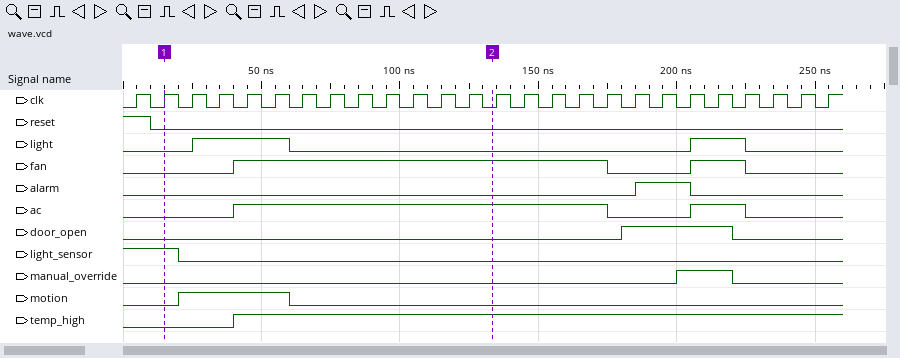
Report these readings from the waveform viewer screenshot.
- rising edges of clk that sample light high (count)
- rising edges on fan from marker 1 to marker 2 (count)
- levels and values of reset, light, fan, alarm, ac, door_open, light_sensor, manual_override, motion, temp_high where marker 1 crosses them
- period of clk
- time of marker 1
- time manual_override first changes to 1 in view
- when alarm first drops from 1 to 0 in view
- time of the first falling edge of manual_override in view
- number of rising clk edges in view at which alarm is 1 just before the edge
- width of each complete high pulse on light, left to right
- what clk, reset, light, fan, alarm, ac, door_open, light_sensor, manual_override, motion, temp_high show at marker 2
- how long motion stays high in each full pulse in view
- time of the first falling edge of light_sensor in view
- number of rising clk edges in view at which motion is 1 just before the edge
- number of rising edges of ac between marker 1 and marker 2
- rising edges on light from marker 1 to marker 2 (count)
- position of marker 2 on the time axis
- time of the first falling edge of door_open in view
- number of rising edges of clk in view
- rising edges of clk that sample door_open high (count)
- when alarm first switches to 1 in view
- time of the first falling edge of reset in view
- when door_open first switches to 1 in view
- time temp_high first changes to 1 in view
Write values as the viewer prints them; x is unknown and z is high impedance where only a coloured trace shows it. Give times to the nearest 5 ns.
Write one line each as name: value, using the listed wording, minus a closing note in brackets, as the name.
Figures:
rising edges of clk that sample light high: 5
rising edges on fan from marker 1 to marker 2: 1
levels and values of reset, light, fan, alarm, ac, door_open, light_sensor, manual_override, motion, temp_high where marker 1 crosses them: reset=0, light=0, fan=0, alarm=0, ac=0, door_open=0, light_sensor=1, manual_override=0, motion=0, temp_high=0
period of clk: 10 ns
time of marker 1: 15 ns
time manual_override first changes to 1 in view: 200 ns
when alarm first drops from 1 to 0 in view: 205 ns
time of the first falling edge of manual_override in view: 220 ns
number of rising clk edges in view at which alarm is 1 just before the edge: 2
width of each complete high pulse on light, left to right: 35 ns, 20 ns
what clk, reset, light, fan, alarm, ac, door_open, light_sensor, manual_override, motion, temp_high show at marker 2: clk=0, reset=0, light=0, fan=1, alarm=0, ac=1, door_open=0, light_sensor=0, manual_override=0, motion=0, temp_high=1
how long motion stays high in each full pulse in view: 40 ns
time of the first falling edge of light_sensor in view: 20 ns
number of rising clk edges in view at which motion is 1 just before the edge: 4
number of rising edges of ac between marker 1 and marker 2: 1
rising edges on light from marker 1 to marker 2: 1
position of marker 2 on the time axis: 135 ns
time of the first falling edge of door_open in view: 220 ns
number of rising edges of clk in view: 26
rising edges of clk that sample door_open high: 4
when alarm first switches to 1 in view: 185 ns
time of the first falling edge of reset in view: 10 ns
when door_open first switches to 1 in view: 180 ns
time temp_high first changes to 1 in view: 40 ns
